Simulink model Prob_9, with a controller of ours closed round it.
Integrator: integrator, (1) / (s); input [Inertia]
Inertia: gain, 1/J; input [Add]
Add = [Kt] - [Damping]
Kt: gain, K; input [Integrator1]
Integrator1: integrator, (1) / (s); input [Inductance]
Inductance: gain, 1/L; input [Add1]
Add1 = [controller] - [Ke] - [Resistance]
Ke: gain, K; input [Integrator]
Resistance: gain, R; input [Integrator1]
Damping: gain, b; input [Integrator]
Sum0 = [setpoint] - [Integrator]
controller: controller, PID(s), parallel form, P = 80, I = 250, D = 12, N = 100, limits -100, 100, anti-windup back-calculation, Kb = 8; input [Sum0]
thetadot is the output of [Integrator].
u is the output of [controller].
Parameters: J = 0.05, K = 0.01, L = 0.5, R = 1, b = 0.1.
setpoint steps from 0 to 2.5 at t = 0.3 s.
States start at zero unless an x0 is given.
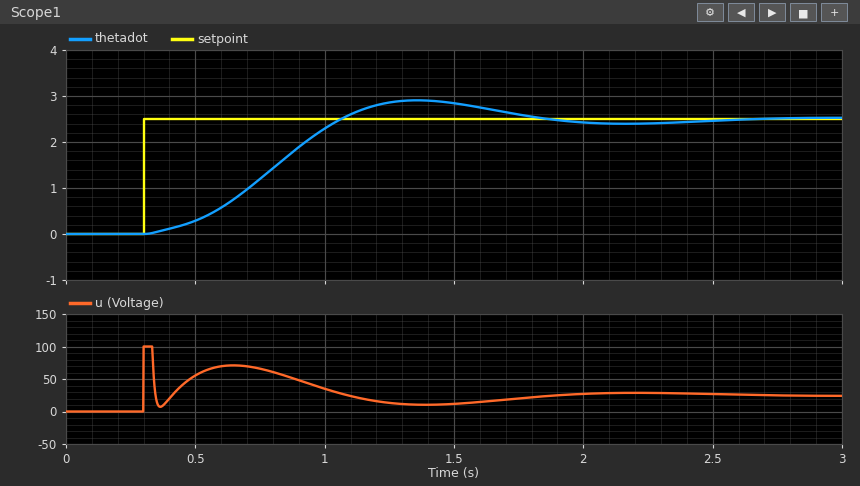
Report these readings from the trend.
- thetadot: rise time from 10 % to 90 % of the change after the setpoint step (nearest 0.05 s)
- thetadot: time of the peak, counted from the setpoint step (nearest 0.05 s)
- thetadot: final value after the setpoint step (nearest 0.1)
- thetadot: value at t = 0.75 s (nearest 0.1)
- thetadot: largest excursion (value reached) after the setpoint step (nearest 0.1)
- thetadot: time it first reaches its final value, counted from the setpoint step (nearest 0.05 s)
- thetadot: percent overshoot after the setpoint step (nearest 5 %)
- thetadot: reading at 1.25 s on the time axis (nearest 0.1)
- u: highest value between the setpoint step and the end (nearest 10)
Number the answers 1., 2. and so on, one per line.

1. 0.50 s
2. 1.05 s
3. 2.5
4. 1.2
5. 2.9
6. 0.75 s
7. 15 %
8. 2.9
9. 100
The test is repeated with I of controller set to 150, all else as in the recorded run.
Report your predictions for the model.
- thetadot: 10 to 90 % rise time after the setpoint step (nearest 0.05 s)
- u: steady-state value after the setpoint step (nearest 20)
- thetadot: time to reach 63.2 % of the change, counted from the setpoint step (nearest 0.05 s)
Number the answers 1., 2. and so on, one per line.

1. 0.85 s
2. 20
3. 0.75 s
